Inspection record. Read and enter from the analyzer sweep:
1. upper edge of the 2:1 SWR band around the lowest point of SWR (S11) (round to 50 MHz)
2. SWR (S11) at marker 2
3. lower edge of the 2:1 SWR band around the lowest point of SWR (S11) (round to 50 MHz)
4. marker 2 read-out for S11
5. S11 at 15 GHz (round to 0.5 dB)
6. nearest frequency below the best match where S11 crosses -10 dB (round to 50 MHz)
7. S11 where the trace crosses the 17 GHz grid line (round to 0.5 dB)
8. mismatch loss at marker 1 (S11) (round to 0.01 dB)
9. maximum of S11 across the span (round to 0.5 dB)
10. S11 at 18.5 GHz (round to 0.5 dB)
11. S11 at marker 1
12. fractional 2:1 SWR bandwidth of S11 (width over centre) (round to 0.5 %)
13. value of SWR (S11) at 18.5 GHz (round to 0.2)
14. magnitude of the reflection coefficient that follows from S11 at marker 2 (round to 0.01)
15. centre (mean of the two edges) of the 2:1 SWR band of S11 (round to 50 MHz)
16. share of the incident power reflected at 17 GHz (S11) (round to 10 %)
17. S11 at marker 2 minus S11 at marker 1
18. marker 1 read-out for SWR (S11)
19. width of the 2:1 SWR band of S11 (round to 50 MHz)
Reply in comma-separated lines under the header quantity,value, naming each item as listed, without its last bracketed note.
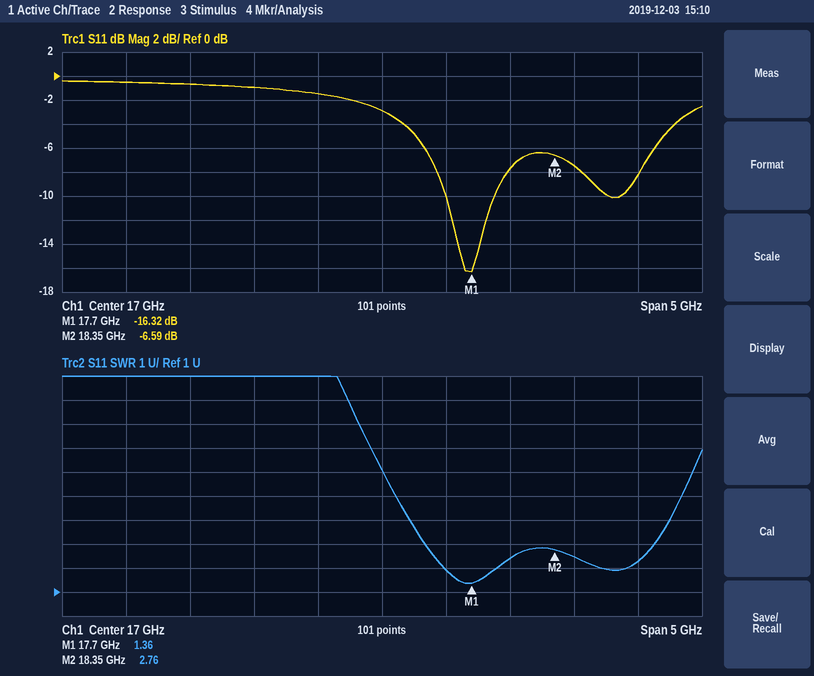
quantity,value
upper edge of the 2:1 SWR band around the lowest point of SWR (S11),17.90 GHz
SWR (S11) at marker 2,2.76
lower edge of the 2:1 SWR band around the lowest point of SWR (S11),17.50 GHz
marker 2 read-out for S11,-6.59 dB
S11 at 15 GHz,-0.5 dB
nearest frequency below the best match where S11 crosses -10 dB,17.50 GHz
S11 where the trace crosses the 17 GHz grid line,-3.0 dB
mismatch loss at marker 1 (S11),0.10 dB
maximum of S11 across the span,-0.5 dB
S11 at 18.5 GHz,-7.5 dB
S11 at marker 1,-16.32 dB
fractional 2:1 SWR bandwidth of S11 (width over centre),2.5 %
value of SWR (S11) at 18.5 GHz,2.4
magnitude of the reflection coefficient that follows from S11 at marker 2,0.47
centre (mean of the two edges) of the 2:1 SWR band of S11,17.70 GHz
share of the incident power reflected at 17 GHz (S11),50 %
S11 at marker 2 minus S11 at marker 1,9.73 dB
marker 1 read-out for SWR,1.36
width of the 2:1 SWR band of S11,400 MHz
